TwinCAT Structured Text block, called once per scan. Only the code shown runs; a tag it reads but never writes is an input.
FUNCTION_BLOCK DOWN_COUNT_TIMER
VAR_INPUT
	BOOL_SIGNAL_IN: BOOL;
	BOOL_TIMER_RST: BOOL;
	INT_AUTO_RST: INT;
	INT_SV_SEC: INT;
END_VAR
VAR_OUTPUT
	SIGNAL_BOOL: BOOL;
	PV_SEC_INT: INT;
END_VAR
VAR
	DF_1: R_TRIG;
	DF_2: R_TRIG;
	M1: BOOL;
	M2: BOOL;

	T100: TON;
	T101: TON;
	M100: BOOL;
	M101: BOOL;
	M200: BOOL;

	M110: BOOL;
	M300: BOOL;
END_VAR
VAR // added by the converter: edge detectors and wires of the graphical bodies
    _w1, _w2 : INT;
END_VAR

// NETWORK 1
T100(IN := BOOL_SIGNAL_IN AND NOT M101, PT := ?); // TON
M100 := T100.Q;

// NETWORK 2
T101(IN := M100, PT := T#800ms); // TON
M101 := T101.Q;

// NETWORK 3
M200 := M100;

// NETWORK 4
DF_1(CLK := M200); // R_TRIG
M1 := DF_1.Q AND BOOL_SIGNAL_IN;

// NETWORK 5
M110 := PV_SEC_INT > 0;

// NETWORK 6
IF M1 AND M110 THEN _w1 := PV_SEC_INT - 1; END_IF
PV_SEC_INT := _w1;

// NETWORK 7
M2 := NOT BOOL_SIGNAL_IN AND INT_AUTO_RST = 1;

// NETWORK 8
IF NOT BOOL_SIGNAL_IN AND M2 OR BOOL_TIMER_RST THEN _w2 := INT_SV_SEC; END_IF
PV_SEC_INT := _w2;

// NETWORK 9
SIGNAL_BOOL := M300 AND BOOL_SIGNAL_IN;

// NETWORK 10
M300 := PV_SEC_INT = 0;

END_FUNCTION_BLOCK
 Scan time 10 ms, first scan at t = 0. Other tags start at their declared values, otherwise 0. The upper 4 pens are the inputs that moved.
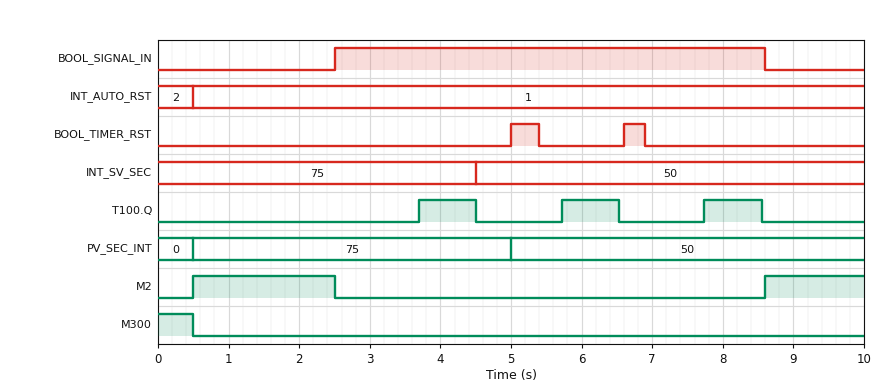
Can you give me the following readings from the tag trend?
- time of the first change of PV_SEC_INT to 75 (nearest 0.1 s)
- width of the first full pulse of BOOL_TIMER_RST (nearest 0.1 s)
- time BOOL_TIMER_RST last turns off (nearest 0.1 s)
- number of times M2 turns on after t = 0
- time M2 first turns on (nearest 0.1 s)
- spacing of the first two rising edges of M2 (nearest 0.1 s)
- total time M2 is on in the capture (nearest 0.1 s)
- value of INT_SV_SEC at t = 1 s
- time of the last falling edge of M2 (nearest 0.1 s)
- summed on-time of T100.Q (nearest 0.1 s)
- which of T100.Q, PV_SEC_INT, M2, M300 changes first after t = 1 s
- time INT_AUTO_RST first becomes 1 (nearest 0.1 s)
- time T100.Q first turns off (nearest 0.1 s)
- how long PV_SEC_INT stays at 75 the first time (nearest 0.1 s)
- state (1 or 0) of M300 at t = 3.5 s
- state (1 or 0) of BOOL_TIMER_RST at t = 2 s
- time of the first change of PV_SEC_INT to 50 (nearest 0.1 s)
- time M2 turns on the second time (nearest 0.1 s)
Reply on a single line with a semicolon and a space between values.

0.5 s; 0.4 s; 6.9 s; 2; 0.5 s; 8.1 s; 3.4 s; 75; 2.5 s; 2.4 s; M2; 0.5 s; 4.5 s; 4.5 s; 0; 0; 5.0 s; 8.6 s
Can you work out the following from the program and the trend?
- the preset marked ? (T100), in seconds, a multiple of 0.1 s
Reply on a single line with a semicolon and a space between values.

1.2 s
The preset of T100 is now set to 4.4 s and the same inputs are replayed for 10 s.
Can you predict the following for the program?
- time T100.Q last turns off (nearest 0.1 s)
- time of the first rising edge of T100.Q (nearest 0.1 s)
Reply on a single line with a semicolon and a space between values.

7.7 s; 6.9 s
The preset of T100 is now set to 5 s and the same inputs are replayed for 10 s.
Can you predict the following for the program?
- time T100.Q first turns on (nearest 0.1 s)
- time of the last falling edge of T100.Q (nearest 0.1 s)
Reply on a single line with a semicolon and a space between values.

7.5 s; 8.3 s
